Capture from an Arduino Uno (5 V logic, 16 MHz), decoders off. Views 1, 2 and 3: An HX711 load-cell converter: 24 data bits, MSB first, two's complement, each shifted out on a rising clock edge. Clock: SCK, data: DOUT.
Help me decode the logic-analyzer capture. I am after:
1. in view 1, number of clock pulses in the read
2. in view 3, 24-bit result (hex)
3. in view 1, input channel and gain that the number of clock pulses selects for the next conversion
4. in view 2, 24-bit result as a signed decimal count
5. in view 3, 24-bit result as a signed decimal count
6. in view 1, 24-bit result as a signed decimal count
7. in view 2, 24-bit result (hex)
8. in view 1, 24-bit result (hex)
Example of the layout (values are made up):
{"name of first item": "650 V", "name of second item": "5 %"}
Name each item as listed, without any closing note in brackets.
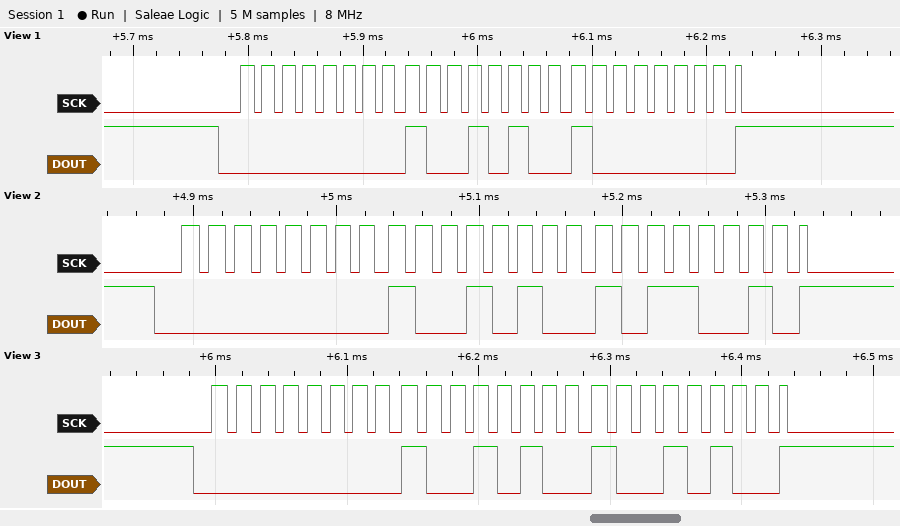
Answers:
{"in view 1, number of clock pulses in the read": "25", "in view 3, 24-bit result": "0x009494", "in view 1, input channel and gain that the number of clock pulses selects for the next conversion": "channel A, gain 128", "in view 2, 24-bit result as a signed decimal count": "38066", "in view 3, 24-bit result as a signed decimal count": "38036", "in view 1, 24-bit result as a signed decimal count": "38016", "in view 2, 24-bit result": "0x0094B2", "in view 1, 24-bit result": "0x009480"}
